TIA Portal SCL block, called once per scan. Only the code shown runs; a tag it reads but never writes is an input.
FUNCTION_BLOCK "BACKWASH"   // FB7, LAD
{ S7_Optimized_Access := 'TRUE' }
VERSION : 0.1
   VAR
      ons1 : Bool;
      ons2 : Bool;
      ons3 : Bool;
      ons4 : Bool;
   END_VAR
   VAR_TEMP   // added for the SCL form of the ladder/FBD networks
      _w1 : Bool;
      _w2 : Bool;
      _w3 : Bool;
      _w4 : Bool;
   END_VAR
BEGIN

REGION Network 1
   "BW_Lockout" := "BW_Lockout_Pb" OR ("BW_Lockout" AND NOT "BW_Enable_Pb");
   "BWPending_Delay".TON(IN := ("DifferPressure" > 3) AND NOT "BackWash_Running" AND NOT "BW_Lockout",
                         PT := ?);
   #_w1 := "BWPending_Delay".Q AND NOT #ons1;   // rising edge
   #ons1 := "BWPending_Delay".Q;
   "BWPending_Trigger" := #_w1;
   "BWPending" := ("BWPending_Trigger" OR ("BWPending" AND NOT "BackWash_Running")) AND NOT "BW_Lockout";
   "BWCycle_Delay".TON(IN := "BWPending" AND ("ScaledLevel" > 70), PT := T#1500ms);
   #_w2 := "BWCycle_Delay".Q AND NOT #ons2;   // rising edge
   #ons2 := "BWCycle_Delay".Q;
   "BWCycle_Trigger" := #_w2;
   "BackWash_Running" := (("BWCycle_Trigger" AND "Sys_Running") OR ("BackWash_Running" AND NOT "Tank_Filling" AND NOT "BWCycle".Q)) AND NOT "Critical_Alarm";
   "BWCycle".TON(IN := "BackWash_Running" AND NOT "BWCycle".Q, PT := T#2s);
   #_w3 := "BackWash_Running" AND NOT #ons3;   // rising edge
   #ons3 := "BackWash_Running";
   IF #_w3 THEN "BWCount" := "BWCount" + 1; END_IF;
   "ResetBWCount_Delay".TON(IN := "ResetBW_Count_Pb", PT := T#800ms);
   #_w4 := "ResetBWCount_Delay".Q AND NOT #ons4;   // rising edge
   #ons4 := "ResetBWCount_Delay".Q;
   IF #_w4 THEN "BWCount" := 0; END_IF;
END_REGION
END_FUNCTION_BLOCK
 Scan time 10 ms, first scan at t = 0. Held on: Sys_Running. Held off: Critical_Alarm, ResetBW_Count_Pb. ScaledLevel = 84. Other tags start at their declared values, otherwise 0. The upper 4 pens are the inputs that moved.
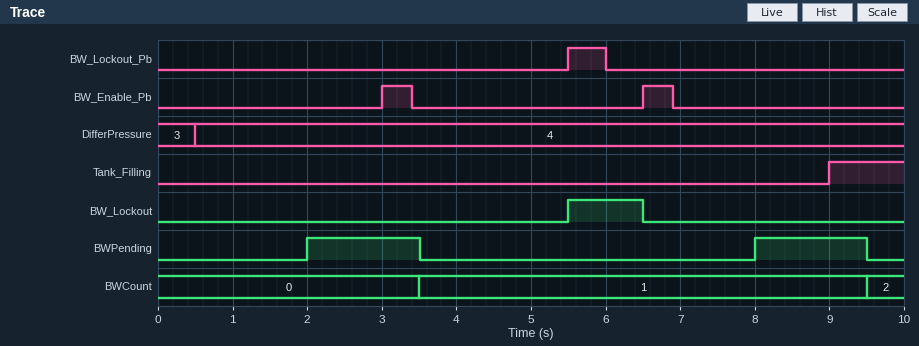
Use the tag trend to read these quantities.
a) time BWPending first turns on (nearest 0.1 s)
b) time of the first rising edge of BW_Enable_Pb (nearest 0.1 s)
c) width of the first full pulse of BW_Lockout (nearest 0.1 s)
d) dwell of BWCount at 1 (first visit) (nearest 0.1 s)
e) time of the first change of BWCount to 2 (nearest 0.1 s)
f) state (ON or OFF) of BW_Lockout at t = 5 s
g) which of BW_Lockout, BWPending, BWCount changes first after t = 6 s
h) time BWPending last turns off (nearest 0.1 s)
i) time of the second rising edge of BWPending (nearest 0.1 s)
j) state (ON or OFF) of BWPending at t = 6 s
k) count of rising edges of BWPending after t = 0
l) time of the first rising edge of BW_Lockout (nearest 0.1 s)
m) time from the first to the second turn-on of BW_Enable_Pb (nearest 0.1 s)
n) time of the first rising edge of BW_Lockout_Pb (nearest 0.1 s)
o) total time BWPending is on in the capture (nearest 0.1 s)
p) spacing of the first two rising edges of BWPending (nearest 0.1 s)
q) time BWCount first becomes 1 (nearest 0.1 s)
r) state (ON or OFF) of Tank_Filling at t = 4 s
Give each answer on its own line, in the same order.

2.0 s
3.0 s
1.0 s
6.0 s
9.5 s
OFF
BW_Lockout
9.5 s
8.0 s
OFF
2
5.5 s
3.5 s
5.5 s
3.0 s
6.0 s
3.5 s
OFF
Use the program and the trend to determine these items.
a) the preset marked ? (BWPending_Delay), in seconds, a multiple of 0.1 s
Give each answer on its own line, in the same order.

1.5 s
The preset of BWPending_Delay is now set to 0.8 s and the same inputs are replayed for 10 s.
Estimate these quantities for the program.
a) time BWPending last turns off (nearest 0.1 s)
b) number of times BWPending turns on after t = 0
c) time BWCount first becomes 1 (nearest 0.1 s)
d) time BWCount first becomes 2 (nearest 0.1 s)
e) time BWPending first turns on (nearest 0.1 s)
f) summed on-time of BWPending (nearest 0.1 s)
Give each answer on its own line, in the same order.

8.8 s
3
2.8 s
8.8 s
1.3 s
3.2 s
